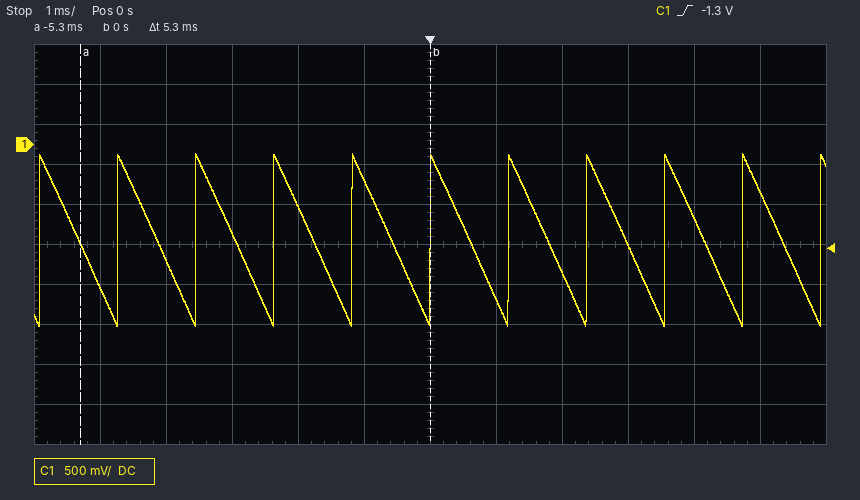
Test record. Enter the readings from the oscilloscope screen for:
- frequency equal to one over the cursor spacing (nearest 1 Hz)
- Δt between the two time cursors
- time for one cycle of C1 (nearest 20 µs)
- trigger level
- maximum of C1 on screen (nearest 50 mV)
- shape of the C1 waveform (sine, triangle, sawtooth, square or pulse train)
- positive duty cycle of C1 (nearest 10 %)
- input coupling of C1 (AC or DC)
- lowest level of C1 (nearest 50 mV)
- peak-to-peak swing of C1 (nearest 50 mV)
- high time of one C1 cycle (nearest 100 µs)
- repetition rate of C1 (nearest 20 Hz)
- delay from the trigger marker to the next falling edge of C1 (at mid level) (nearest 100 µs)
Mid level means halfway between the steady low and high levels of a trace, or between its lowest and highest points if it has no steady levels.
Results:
189 Hz
5.3 ms
1.18 ms
-1.3 V
-100 mV
sawtooth
50 %
DC
-2.25 V
2.15 V
600 µs
840 Hz
600 µs
